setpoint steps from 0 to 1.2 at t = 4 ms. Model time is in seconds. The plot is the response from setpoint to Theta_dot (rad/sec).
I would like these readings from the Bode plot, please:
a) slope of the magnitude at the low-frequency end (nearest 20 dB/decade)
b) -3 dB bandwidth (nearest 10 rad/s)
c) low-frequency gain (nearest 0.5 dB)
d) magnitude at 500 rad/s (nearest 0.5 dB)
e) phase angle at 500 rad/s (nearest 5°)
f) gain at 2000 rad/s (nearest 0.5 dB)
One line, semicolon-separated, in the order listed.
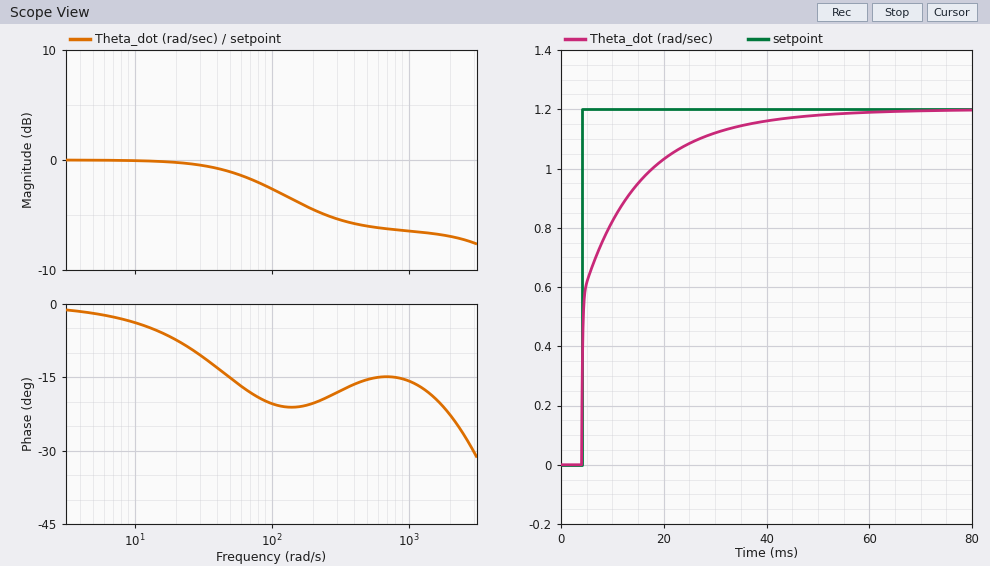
0 dB/decade; 120 rad/s; 0.0 dB; -6.0 dB; -15°; -7.0 dB
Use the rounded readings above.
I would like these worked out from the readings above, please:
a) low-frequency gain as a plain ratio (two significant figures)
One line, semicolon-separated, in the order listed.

1.0
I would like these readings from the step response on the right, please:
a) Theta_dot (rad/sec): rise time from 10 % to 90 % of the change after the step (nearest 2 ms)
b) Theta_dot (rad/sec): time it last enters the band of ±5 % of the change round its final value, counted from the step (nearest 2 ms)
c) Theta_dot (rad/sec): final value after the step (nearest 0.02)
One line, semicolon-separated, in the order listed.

20 ms; 30 ms; 1.20
